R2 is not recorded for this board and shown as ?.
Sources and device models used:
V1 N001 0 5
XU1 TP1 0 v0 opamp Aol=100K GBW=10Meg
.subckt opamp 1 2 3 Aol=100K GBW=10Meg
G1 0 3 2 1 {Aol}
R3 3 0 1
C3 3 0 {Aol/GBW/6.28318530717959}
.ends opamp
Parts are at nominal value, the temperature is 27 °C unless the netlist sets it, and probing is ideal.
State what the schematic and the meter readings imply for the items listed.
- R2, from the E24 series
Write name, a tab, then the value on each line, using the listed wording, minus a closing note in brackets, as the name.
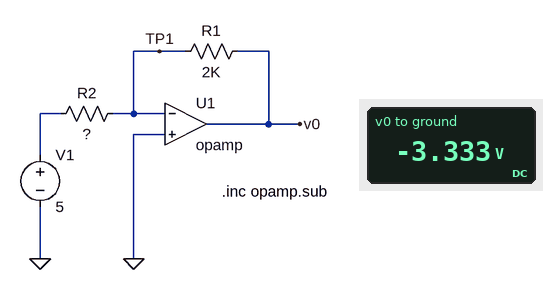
R2, from the E24 series	3 kΩ
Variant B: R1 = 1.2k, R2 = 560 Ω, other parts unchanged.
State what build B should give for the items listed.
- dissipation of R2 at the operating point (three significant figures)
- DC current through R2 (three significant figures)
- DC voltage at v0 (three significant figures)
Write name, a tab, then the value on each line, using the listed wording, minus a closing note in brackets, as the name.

dissipation of R2 at the operating point	44.6 mW
DC current through R2	8.93 mA
DC voltage at v0	-10.7 V
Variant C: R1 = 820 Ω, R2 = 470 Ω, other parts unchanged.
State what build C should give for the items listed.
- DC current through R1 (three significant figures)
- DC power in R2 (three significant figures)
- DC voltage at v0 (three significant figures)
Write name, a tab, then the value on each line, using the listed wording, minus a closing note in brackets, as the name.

DC current through R1	10.6 mA
DC power in R2	53.2 mW
DC voltage at v0	-8.72 V
